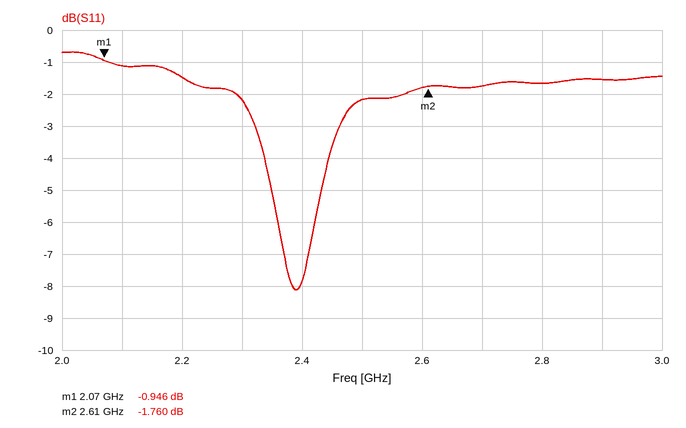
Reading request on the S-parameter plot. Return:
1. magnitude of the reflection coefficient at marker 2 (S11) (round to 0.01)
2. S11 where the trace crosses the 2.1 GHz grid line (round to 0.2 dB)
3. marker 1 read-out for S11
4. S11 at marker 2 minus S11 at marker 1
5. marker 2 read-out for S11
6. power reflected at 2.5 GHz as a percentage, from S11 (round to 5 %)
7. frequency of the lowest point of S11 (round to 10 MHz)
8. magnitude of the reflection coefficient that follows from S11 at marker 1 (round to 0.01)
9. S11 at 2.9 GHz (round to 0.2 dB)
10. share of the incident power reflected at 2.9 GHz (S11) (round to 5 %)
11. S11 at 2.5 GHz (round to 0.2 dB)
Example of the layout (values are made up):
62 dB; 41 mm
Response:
0.82; -1.2 dB; -0.946 dB; -0.814 dB; -1.760 dB; 60 %; 2.39 GHz; 0.90; -1.6 dB; 70 %; -2.2 dB
